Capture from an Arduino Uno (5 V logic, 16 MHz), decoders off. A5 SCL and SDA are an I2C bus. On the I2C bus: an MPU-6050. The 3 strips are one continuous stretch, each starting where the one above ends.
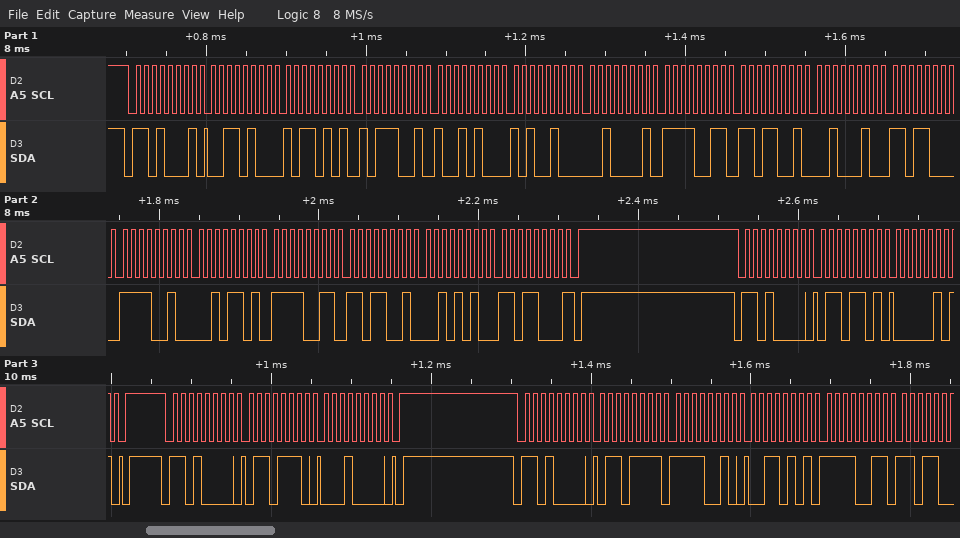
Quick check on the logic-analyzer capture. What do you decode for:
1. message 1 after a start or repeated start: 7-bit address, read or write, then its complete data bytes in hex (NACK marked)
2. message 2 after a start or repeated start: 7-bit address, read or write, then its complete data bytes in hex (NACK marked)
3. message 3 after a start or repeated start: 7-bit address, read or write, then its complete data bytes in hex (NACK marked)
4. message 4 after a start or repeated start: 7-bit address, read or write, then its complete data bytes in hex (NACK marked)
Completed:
0x68 read: 34 B5 B9 94 A4 21 F3 D9 22 D8 F2 2D F3 D9 2A D8 NACK
0x68 write: 6D 05
0x68 write: 6E 10
0x68 write: 6F F2 35 F3
